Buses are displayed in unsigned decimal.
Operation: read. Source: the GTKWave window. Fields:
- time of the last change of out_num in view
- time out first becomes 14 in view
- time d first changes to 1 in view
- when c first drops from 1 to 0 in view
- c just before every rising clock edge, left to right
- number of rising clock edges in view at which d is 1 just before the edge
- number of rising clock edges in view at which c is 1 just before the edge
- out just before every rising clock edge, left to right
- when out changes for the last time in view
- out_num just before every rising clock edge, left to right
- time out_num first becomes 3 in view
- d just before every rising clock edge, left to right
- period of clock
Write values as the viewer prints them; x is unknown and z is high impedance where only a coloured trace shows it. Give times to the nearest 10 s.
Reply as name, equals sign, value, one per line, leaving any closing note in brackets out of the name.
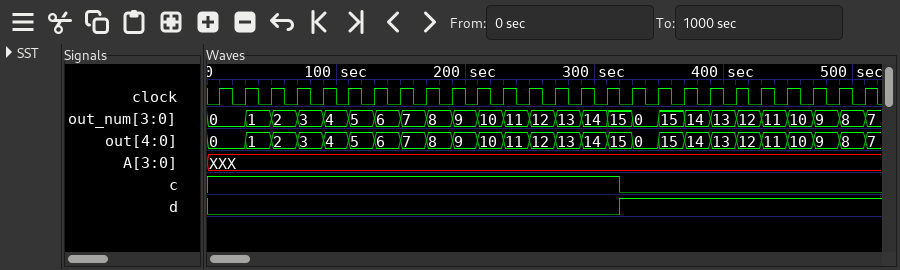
time of the last change of out_num in view = 510 s
time out first becomes 14 in view = 290 s
time d first changes to 1 in view = 320 s
when c first drops from 1 to 0 in view = 320 s
c just before every rising clock edge, left to right = 1 1 1 1 1 1 1 1 1 1 1 1 1 1 1 1 0 0 0 0 0 0 0 0 0 0
number of rising clock edges in view at which d is 1 just before the edge = 10
number of rising clock edges in view at which c is 1 just before the edge = 16
out just before every rising clock edge, left to right = 0, 0, 1, 2, 3, 4, 5, 6, 7, 8, 9, 10, 11, 12, 13, 14, 15, 0, 15, 14, 13, 12, 11, 10, 9, 8
when out changes for the last time in view = 510 s
out_num just before every rising clock edge, left to right = 0, 0, 1, 2, 3, 4, 5, 6, 7, 8, 9, 10, 11, 12, 13, 14, 15, 0, 15, 14, 13, 12, 11, 10, 9, 8
time out_num first becomes 3 in view = 70 s
d just before every rising clock edge, left to right = 0 0 0 0 0 0 0 0 0 0 0 0 0 0 0 0 1 1 1 1 1 1 1 1 1 1
period of clock = 20 s
